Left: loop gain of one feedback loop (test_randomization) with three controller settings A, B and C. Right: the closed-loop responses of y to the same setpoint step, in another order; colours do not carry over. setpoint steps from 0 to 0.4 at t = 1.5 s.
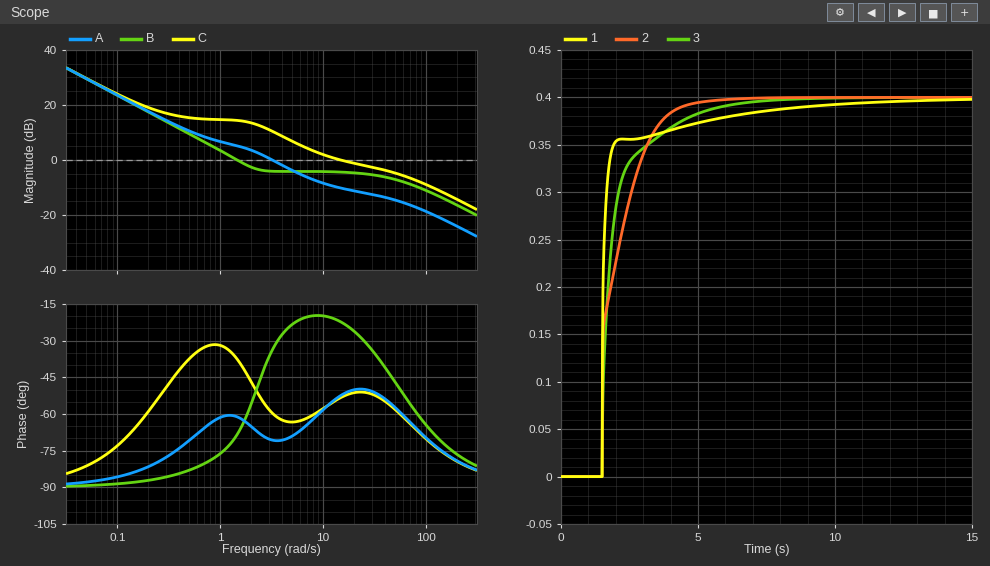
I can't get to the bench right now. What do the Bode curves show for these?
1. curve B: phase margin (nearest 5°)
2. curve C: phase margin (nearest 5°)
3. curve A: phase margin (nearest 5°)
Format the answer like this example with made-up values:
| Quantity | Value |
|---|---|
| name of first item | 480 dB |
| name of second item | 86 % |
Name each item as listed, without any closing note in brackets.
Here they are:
| Quantity | Value |
|---|---|
| curve B: phase margin | 110° |
| curve C: phase margin | 125° |
| curve A: phase margin | 110° |
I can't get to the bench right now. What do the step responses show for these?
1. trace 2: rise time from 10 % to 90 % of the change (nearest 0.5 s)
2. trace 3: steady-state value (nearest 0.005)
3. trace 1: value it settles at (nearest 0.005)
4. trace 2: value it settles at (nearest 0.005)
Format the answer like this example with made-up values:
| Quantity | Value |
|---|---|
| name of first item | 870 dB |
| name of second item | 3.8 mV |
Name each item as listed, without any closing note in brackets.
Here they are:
| Quantity | Value |
|---|---|
| trace 2: rise time from 10 % to 90 % of the change | 2.0 s |
| trace 3: steady-state value | 0.400 |
| trace 1: value it settles at | 0.400 |
| trace 2: value it settles at | 0.400 |
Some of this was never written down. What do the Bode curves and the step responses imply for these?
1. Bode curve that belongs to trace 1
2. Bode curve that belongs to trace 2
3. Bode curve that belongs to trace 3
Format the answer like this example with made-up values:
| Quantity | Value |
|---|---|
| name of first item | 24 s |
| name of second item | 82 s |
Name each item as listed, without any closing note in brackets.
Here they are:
| Quantity | Value |
|---|---|
| Bode curve that belongs to trace 1 | C |
| Bode curve that belongs to trace 2 | B |
| Bode curve that belongs to trace 3 | A |
